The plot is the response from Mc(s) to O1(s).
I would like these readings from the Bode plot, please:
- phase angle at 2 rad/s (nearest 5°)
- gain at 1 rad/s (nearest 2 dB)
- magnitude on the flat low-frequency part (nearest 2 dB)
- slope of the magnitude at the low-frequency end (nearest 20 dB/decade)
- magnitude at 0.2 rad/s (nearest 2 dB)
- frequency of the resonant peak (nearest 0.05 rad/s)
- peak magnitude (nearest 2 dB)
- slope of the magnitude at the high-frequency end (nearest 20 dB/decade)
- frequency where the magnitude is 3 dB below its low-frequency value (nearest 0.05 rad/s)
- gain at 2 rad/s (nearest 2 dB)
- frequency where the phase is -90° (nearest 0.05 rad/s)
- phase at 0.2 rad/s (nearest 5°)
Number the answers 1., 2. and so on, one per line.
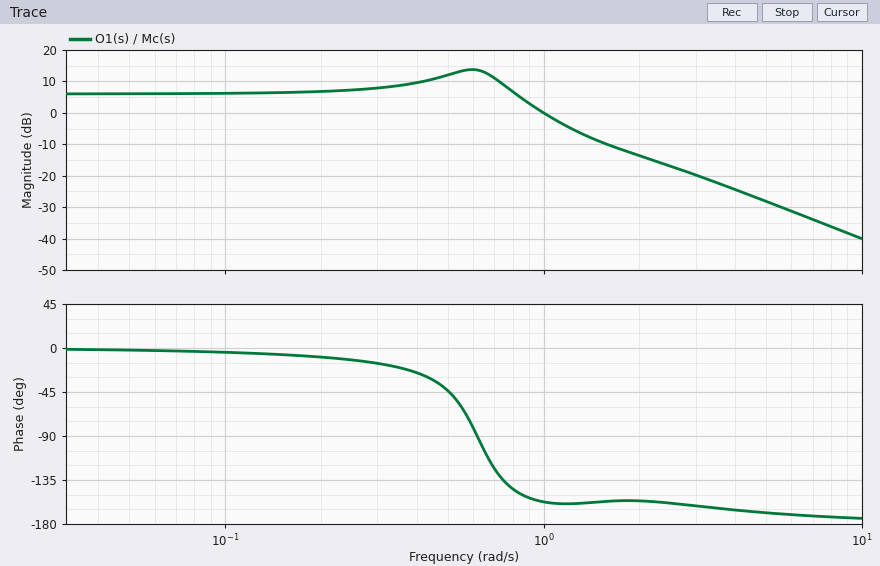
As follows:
1. -155°
2. 0 dB
3. 6 dB
4. 0 dB/decade
5. 6 dB
6. 0.60 rad/s
7. 14 dB
8. -40 dB/decade
9. 0.90 rad/s
10. -14 dB
11. 0.60 rad/s
12. -10°
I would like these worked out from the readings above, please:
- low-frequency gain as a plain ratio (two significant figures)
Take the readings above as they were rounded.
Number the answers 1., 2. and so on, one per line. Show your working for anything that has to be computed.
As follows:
1. 10^(6 / 20) = 2.0
